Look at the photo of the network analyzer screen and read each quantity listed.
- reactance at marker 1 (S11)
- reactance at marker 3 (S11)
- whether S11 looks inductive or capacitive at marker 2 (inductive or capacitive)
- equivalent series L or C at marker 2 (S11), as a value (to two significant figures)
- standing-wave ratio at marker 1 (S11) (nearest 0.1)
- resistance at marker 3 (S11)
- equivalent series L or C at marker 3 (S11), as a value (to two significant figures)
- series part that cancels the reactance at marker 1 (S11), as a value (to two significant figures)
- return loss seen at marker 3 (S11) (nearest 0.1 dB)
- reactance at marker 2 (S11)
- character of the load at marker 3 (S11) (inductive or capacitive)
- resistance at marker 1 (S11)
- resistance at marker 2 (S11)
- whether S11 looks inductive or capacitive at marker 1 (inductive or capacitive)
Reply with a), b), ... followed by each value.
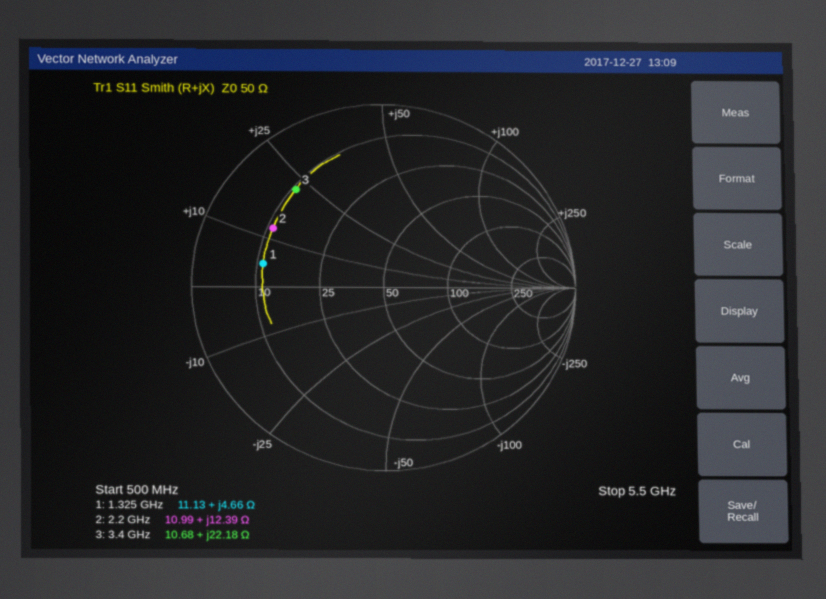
a) +4.66 Ω
b) +22.18 Ω
c) inductive
d) 900 pH
e) 4.5
f) 10.68 Ω
g) 1.0 nH
h) 26 pF
i) 3.1 dB
j) +12.39 Ω
k) inductive
l) 11.13 Ω
m) 10.99 Ω
n) inductive
